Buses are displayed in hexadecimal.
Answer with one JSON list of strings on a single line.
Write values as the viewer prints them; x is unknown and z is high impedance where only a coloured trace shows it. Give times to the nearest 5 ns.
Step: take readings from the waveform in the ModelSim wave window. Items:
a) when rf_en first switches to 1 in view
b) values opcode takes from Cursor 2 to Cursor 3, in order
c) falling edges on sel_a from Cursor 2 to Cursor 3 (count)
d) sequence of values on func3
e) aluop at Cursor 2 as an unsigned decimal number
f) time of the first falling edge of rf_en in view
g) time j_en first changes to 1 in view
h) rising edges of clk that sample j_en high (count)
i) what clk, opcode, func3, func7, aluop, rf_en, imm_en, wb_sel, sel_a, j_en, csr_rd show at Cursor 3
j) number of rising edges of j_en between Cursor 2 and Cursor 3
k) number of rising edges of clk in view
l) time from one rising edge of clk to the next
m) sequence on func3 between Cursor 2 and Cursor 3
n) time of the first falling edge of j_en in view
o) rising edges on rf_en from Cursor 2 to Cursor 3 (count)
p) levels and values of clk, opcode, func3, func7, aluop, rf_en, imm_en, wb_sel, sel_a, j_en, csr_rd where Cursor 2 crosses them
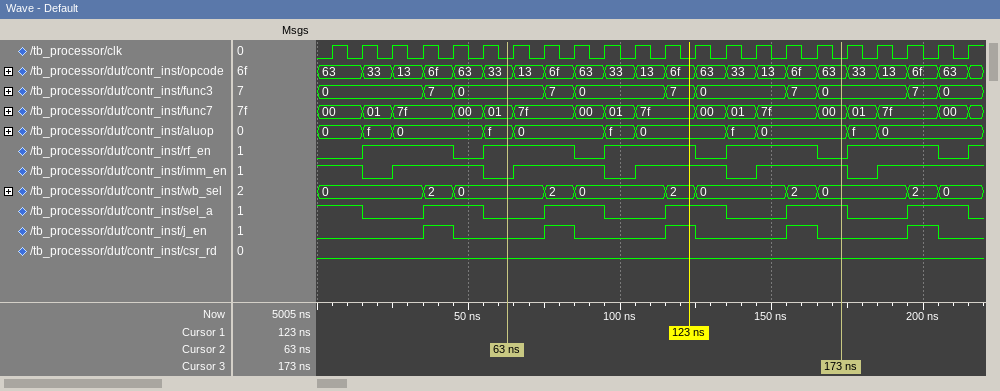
["15 ns", "33, 13, 6f, 63, 33, 13, 6f, 63, 33, 13, 6f, 63", "2", "0, 7, 0, 7, 0, 7, 0, 7, 0, 7, 0", "15", "45 ns", "35 ns", "5", "clk=0, opcode=63, func3=0, func7=00, aluop=0, rf_en=0, imm_en=1, wb_sel=0, sel_a=1, j_en=0, csr_rd=0", "3", "22", "10 ns", "0, 7, 0, 7, 0, 7, 0", "45 ns", "2", "clk=0, opcode=33, func3=0, func7=01, aluop=f, rf_en=1, imm_en=0, wb_sel=0, sel_a=0, j_en=0, csr_rd=0"]
